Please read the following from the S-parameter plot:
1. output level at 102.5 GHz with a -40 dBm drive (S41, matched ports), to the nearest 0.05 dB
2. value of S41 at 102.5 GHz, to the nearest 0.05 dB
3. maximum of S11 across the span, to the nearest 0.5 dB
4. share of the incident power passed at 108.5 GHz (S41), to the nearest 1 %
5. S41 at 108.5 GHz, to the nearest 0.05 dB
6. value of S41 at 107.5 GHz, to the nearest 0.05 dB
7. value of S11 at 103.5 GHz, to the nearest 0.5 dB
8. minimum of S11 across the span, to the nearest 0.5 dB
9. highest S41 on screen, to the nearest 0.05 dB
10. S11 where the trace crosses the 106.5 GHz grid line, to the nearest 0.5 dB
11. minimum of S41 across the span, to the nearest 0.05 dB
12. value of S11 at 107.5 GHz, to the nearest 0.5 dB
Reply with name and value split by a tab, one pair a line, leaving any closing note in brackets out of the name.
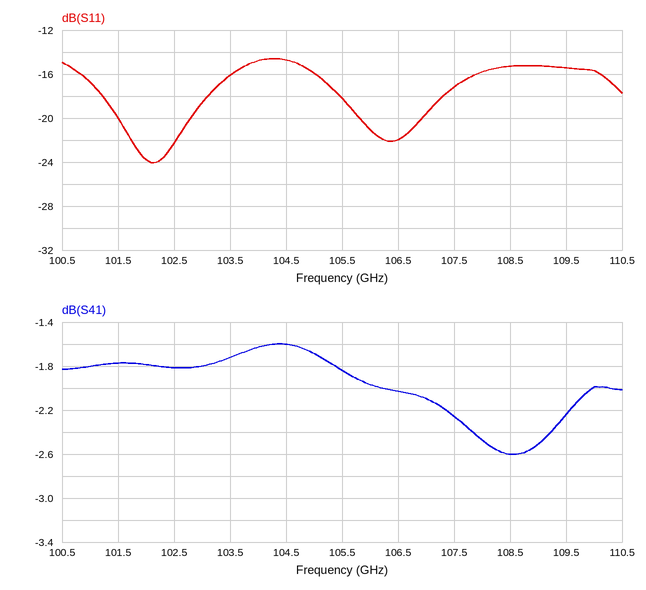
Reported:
output level at 102.5 GHz with a -40 dBm drive (S41, matched ports), to the nearest 0.05 dB	-41.80 dBm
value of S41 at 102.5 GHz, to the nearest 0.05 dB	-1.80 dB
maximum of S11 across the span, to the nearest 0.5 dB	-14.5 dB
share of the incident power passed at 108.5 GHz (S41), to the nearest 1 %	55 %
S41 at 108.5 GHz, to the nearest 0.05 dB	-2.60 dB
value of S41 at 107.5 GHz, to the nearest 0.05 dB	-2.25 dB
value of S11 at 103.5 GHz, to the nearest 0.5 dB	-16.0 dB
minimum of S11 across the span, to the nearest 0.5 dB	-24.0 dB
highest S41 on screen, to the nearest 0.05 dB	-1.60 dB
S11 where the trace crosses the 106.5 GHz grid line, to the nearest 0.5 dB	-22.0 dB
minimum of S41 across the span, to the nearest 0.05 dB	-2.60 dB
value of S11 at 107.5 GHz, to the nearest 0.5 dB	-17.0 dB
